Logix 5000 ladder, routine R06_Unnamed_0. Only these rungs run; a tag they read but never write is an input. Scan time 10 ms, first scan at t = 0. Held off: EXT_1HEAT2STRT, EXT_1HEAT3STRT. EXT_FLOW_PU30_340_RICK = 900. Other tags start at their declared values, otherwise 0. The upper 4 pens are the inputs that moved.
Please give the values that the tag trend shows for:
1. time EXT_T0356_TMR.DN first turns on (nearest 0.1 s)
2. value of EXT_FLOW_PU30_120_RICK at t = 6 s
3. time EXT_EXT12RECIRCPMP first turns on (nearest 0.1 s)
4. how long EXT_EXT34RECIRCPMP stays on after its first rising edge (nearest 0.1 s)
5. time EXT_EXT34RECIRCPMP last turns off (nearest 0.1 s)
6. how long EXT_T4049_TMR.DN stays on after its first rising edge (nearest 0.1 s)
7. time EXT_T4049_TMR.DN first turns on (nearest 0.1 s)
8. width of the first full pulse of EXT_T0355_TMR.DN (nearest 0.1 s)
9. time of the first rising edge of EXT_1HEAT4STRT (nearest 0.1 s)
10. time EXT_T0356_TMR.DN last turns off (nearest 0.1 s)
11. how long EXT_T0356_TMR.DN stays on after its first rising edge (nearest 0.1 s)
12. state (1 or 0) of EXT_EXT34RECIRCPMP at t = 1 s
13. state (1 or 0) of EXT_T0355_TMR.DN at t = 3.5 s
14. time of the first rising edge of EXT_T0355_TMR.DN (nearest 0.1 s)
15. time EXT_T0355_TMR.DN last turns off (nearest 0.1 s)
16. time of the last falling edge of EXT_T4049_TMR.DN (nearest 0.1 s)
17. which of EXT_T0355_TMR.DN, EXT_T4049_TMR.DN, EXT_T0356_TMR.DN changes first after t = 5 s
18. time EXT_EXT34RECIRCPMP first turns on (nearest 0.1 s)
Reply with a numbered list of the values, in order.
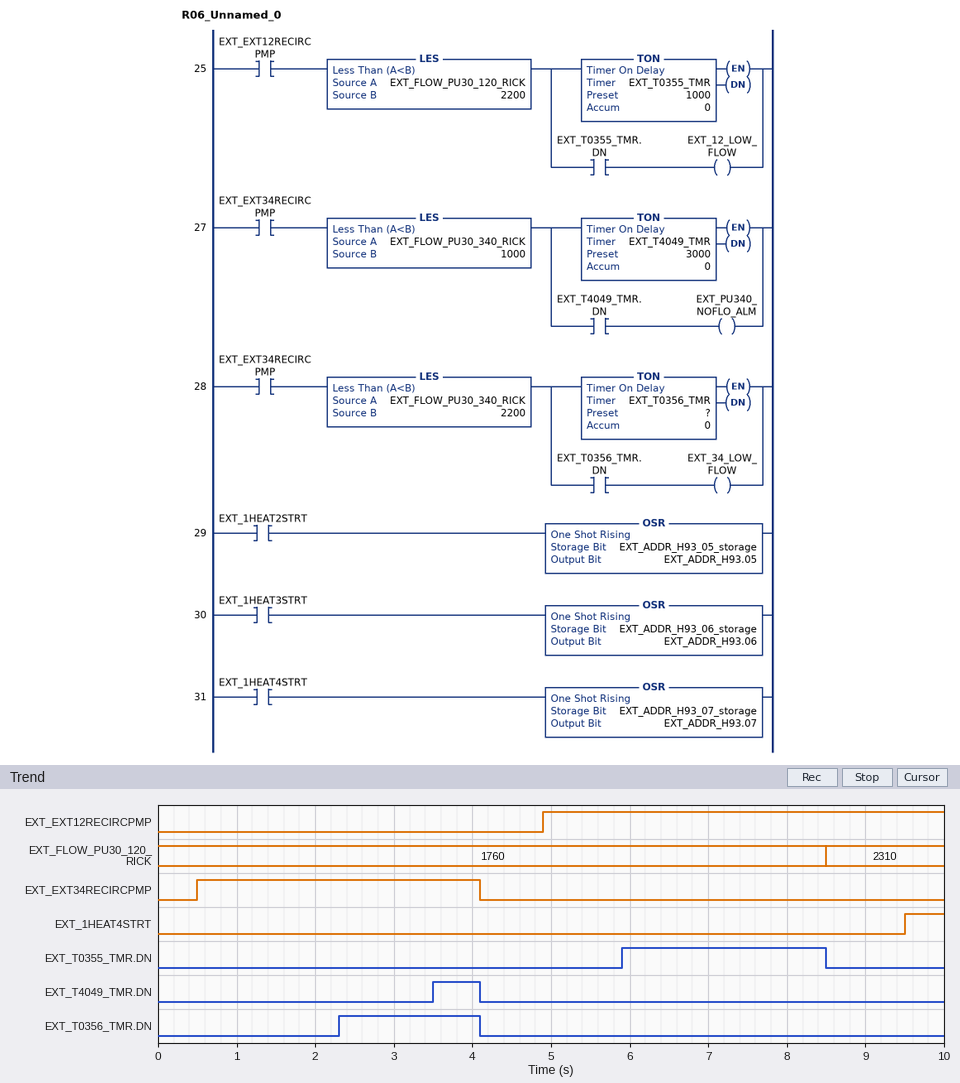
1. 2.3 s
2. 1760
3. 4.9 s
4. 3.6 s
5. 4.1 s
6. 0.6 s
7. 3.5 s
8. 2.6 s
9. 9.5 s
10. 4.1 s
11. 1.8 s
12. 1
13. 0
14. 5.9 s
15. 8.5 s
16. 4.1 s
17. EXT_T0355_TMR.DN
18. 0.5 s
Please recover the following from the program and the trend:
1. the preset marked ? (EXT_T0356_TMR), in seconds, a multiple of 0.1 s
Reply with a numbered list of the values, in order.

1. 1.8 s
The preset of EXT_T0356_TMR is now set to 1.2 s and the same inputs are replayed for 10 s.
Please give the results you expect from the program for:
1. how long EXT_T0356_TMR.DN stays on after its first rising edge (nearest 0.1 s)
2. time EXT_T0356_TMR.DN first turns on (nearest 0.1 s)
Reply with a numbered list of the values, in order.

1. 2.4 s
2. 1.7 s
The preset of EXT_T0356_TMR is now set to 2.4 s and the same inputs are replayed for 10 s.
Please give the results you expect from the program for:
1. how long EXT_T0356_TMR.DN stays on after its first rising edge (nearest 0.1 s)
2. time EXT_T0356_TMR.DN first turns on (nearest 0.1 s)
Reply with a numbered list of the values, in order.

1. 1.2 s
2. 2.9 s
